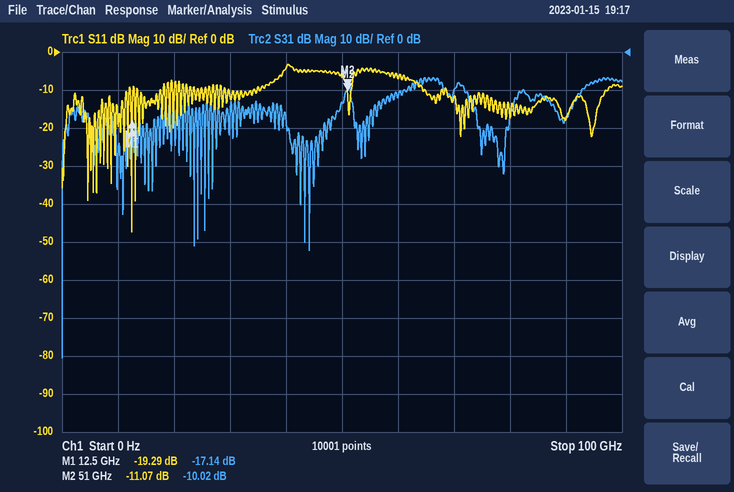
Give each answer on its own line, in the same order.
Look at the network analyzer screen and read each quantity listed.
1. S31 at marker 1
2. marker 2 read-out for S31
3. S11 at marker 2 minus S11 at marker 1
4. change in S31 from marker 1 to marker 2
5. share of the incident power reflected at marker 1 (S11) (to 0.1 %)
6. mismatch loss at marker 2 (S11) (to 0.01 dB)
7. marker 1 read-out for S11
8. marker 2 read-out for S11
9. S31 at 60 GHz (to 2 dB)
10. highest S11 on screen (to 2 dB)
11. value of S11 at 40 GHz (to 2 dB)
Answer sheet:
-17.14 dB
-10.02 dB
8.22 dB
7.12 dB
1.2 %
0.35 dB
-19.29 dB
-11.07 dB
-12 dB
-4 dB
-4 dB
